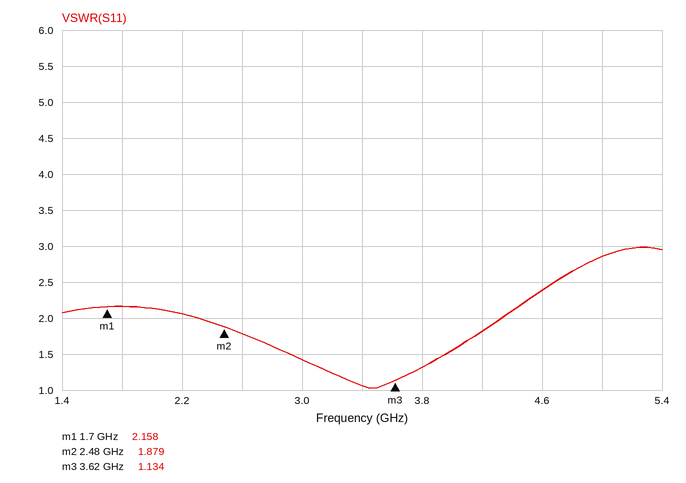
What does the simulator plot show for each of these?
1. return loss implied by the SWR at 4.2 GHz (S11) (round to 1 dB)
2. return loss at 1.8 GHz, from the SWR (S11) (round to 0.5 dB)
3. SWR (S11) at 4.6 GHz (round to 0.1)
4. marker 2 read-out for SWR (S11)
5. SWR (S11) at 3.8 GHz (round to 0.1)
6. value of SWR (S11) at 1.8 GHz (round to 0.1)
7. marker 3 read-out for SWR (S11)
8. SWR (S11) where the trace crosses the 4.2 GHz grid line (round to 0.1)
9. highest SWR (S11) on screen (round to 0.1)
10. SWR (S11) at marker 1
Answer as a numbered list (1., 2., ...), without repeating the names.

1. 11 dB
2. 8.5 dB
3. 2.4
4. 1.879
5. 1.3
6. 2.2
7. 1.134
8. 1.8
9. 3.0
10. 2.158
